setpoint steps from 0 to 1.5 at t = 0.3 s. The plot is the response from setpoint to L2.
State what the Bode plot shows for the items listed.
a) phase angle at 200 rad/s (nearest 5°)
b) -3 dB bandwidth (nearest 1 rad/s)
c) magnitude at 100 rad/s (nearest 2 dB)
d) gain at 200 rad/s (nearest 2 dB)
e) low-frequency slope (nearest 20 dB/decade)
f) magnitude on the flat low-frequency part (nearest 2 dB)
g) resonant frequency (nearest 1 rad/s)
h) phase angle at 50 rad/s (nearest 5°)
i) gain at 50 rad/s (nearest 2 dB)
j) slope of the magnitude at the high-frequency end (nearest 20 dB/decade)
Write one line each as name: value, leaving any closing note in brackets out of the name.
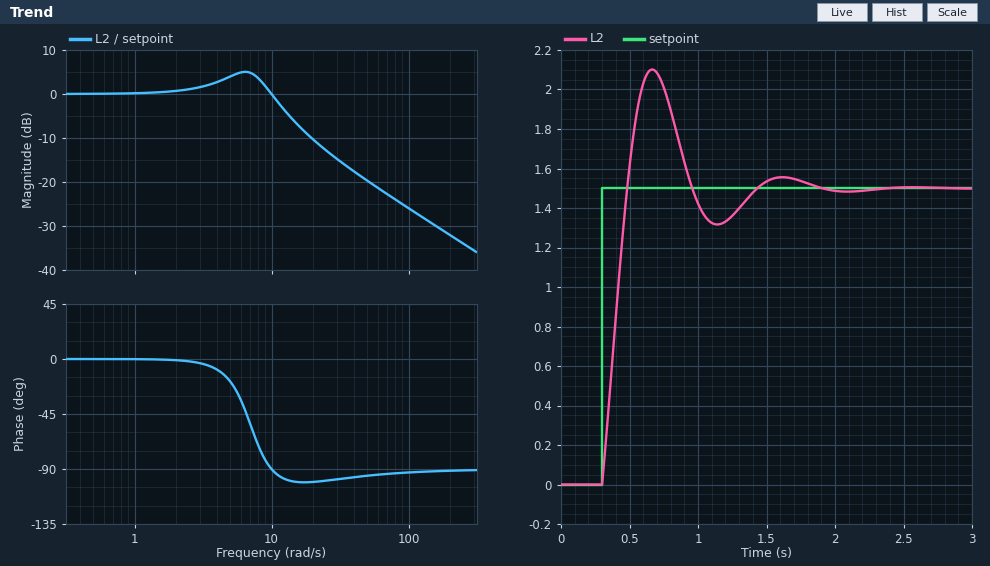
phase angle at 200 rad/s: -90°
-3 dB bandwidth: 12 rad/s
magnitude at 100 rad/s: -26 dB
gain at 200 rad/s: -32 dB
low-frequency slope: 0 dB/decade
magnitude on the flat low-frequency part: 0 dB
resonant frequency: 6 rad/s
phase angle at 50 rad/s: -95°
gain at 50 rad/s: -20 dB
slope of the magnitude at the high-frequency end: -20 dB/decade
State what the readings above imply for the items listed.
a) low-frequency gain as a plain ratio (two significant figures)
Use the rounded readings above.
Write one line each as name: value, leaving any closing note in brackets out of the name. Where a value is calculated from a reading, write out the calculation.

low-frequency gain as a plain ratio: 10^(0 / 20) = 1.0
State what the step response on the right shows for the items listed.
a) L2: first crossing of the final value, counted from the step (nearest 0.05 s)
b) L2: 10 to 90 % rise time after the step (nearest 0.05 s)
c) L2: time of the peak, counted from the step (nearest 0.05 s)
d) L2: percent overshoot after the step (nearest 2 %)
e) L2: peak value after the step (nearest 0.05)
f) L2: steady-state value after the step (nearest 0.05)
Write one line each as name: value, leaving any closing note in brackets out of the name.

L2: first crossing of the final value, counted from the step: 0.20 s
L2: 10 to 90 % rise time after the step: 0.15 s
L2: time of the peak, counted from the step: 0.35 s
L2: percent overshoot after the step: 40 %
L2: peak value after the step: 2.10
L2: steady-state value after the step: 1.50
